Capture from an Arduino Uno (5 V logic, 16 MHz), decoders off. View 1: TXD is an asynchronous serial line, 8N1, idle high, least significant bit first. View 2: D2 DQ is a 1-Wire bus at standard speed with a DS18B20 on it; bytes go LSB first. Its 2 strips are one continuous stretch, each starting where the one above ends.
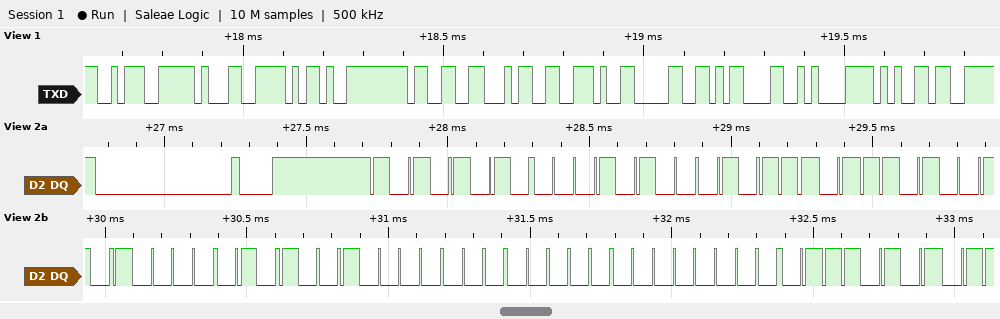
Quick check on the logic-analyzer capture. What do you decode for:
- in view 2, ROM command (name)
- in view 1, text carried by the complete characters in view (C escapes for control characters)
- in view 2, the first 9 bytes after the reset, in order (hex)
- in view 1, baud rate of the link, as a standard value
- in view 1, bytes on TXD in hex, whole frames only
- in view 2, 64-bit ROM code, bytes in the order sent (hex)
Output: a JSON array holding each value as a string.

["Match ROM", "\":1-34.0\\r\\ne\"", "55 28 BA 4B 41 09 00 00 AE", "57600 baud", "3A 31 2D 33 34 2E 30 0D 0A 65", "28 BA 4B 41 09 00 00 AE"]
